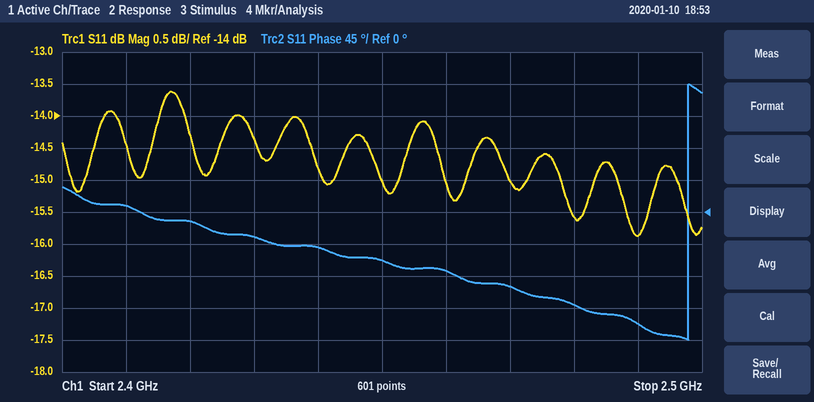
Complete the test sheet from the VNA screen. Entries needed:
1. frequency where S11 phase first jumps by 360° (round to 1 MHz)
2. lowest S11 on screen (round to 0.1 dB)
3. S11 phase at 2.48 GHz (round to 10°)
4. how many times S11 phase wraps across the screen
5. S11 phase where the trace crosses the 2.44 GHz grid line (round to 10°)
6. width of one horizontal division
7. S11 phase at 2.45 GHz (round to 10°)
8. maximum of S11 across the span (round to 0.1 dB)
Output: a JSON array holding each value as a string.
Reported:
["2.498 GHz", "-15.9 dB", "-130°", "1", "-50°", "10 MHz", "-70°", "-13.6 dB"]
